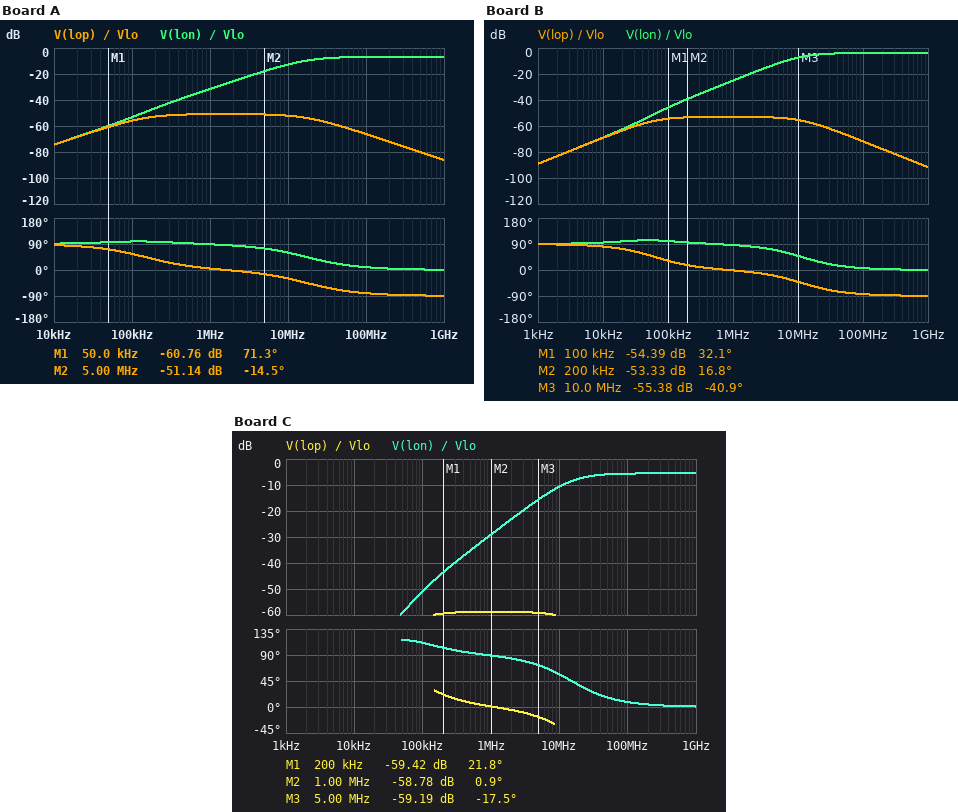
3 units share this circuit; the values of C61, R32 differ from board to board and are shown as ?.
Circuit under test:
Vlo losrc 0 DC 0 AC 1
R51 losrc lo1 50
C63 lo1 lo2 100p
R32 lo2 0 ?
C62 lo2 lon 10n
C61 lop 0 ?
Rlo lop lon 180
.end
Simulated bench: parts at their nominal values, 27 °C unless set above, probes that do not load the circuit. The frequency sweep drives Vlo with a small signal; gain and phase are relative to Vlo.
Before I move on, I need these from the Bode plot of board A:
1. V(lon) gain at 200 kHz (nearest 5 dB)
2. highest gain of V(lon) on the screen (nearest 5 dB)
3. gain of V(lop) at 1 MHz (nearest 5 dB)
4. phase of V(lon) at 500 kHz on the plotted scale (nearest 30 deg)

-45 dB
-5 dB
-50 dB
90 deg
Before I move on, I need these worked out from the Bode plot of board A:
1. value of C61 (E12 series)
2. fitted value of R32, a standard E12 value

8.2 nF
56 Ω
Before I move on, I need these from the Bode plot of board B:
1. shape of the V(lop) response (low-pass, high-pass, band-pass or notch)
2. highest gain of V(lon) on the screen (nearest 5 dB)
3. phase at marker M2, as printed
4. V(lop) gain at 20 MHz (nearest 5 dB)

band-pass
-5 dB
16.8 deg
-60 dB
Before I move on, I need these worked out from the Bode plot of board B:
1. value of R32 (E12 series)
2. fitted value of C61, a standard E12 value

180 Ω
22 nF
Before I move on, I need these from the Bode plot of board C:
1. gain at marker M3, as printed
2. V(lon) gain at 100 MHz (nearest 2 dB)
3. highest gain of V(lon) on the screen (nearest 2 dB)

-59.19 dB
-6 dB
-6 dB
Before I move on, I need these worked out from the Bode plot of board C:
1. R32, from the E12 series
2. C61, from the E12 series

82 Ω
27 nF
